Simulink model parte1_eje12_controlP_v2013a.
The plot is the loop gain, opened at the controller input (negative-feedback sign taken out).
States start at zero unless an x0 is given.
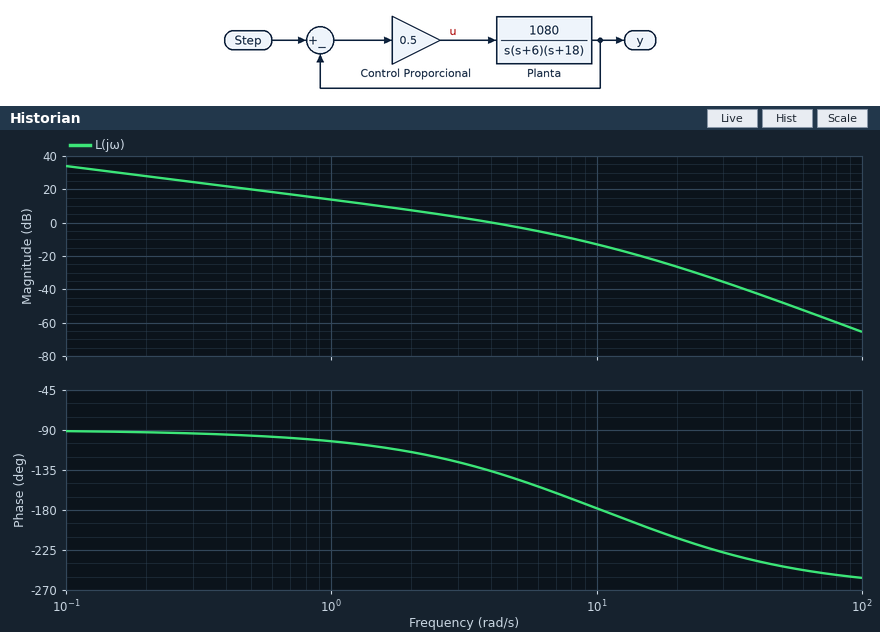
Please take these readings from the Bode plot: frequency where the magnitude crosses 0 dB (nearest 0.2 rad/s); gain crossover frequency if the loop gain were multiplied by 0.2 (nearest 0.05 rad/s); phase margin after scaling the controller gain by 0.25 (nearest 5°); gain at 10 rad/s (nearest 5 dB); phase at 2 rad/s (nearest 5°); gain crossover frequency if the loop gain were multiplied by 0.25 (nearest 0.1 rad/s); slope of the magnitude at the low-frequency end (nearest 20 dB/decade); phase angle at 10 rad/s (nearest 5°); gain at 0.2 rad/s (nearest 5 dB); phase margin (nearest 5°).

4.0 rad/s
1.00 rad/s
75°
-15 dB
-115°
1.2 rad/s
-20 dB/decade
-180°
30 dB
45°
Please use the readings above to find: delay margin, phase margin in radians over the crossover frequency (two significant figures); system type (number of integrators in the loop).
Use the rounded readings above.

0.20 s
1
